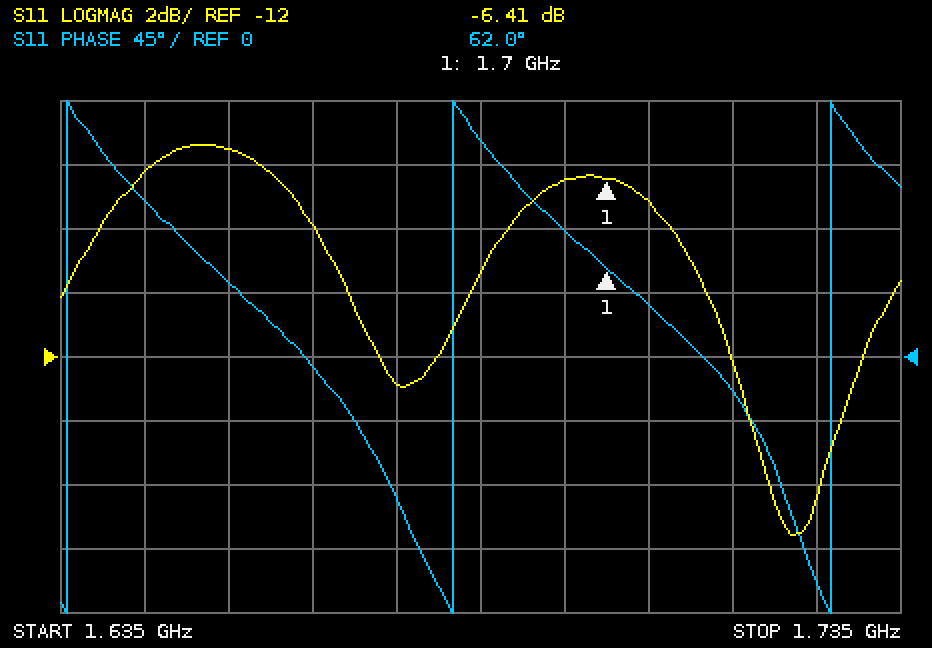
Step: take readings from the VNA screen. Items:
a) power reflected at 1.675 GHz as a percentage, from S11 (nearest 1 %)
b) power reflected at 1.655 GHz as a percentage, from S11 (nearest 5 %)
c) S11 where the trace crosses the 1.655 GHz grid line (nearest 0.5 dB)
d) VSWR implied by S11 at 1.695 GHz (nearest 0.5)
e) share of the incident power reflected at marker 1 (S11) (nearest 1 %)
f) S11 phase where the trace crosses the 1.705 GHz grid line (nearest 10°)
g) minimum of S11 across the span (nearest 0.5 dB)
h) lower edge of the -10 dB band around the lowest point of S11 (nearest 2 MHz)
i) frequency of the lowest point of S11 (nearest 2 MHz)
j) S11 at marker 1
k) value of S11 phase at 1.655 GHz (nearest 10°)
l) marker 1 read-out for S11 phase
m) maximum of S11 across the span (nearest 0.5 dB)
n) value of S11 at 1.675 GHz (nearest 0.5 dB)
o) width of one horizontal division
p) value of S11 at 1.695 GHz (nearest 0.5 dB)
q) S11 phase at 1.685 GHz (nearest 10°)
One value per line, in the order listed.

5 %
30 %
-5.5 dB
3.0
23 %
40°
-17.5 dB
1.712 GHz
1.722 GHz
-6.41 dB
50°
62.0°
-5.5 dB
-13.0 dB
10 MHz
-6.5 dB
150°
